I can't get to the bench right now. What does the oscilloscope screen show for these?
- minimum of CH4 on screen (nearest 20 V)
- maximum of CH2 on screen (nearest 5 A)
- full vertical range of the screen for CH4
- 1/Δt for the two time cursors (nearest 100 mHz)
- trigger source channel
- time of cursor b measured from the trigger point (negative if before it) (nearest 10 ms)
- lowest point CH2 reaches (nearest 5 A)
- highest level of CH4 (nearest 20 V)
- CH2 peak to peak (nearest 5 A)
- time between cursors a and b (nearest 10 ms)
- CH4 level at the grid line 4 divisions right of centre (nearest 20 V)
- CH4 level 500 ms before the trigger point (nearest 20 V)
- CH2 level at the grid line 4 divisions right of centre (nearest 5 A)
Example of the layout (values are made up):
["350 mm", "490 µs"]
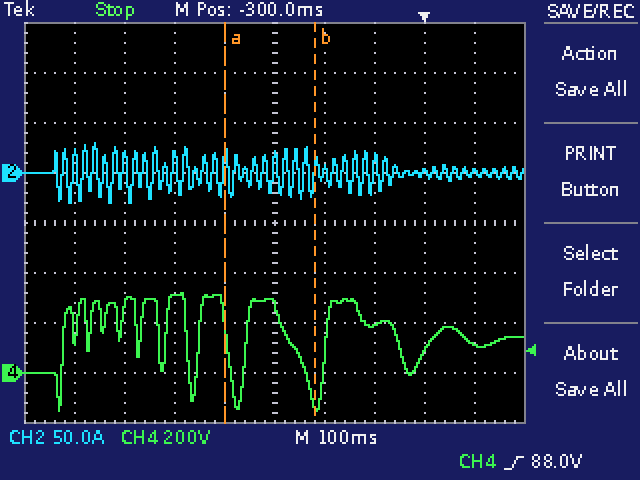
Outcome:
["-160 V", "30 A", "1.6 kV", "5.6 Hz", "CH4", "-220 ms", "-30 A", "320 V", "60 A", "180 ms", "120 V", "300 V", "0 A"]
